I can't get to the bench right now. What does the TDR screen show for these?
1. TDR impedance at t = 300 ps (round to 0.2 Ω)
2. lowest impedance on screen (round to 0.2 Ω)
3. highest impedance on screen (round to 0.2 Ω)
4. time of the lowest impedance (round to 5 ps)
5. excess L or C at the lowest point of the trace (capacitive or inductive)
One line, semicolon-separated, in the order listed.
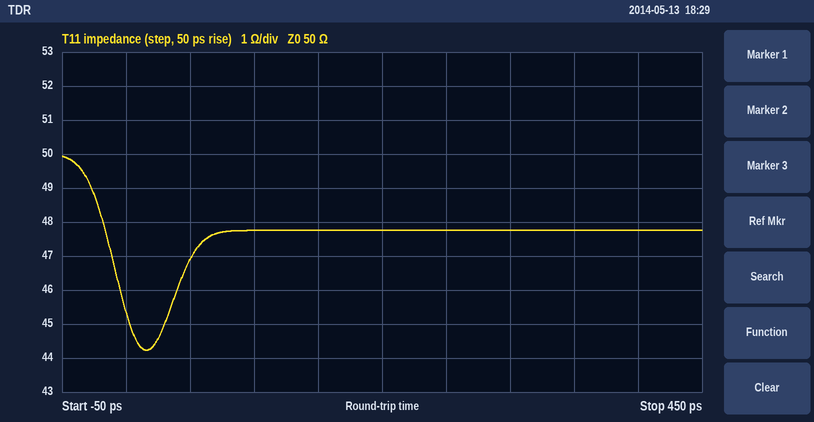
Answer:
47.8 Ω; 44.2 Ω; 50.0 Ω; 15 ps; capacitive
